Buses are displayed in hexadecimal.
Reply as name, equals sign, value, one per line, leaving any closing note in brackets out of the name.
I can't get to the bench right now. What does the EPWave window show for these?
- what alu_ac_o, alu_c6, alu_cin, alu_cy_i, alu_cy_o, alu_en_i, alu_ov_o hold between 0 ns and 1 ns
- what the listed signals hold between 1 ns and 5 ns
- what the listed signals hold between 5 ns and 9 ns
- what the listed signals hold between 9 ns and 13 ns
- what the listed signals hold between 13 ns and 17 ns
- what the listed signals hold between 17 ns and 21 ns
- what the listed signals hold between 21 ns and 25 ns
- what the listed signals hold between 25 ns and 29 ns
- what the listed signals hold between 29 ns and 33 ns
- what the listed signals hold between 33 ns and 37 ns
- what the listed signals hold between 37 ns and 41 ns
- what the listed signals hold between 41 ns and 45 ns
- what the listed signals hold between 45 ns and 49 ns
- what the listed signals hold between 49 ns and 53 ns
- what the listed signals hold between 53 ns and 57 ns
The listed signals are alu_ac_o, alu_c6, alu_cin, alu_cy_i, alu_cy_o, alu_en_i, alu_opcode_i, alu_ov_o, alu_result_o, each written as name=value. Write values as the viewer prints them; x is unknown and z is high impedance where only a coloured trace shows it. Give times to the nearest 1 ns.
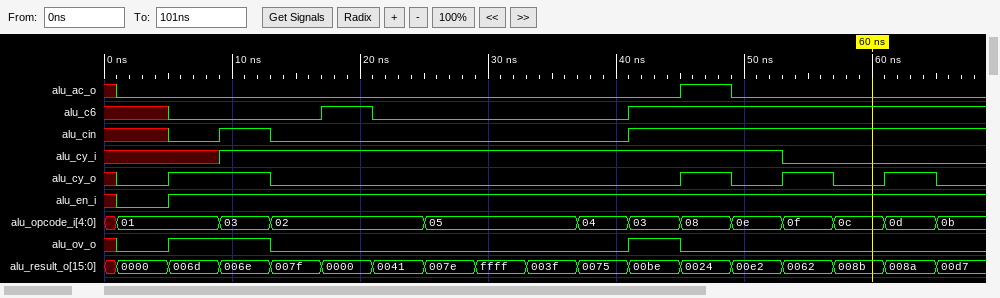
what alu_ac_o, alu_c6, alu_cin, alu_cy_i, alu_cy_o, alu_en_i, alu_ov_o hold between 0 ns and 1 ns = alu_ac_o=x, alu_c6=x, alu_cin=x, alu_cy_i=x, alu_cy_o=x, alu_en_i=x, alu_ov_o=x
what the listed signals hold between 1 ns and 5 ns = alu_ac_o=0, alu_c6=x, alu_cin=x, alu_cy_i=x, alu_cy_o=0, alu_en_i=0, alu_opcode_i=01, alu_ov_o=0, alu_result_o=0000
what the listed signals hold between 5 ns and 9 ns = alu_ac_o=0, alu_c6=0, alu_cin=0, alu_cy_i=x, alu_cy_o=1, alu_en_i=1, alu_opcode_i=01, alu_ov_o=1, alu_result_o=006d
what the listed signals hold between 9 ns and 13 ns = alu_ac_o=0, alu_c6=0, alu_cin=1, alu_cy_i=1, alu_cy_o=1, alu_en_i=1, alu_opcode_i=03, alu_ov_o=1, alu_result_o=006e
what the listed signals hold between 13 ns and 17 ns = alu_ac_o=0, alu_c6=0, alu_cin=0, alu_cy_i=1, alu_cy_o=0, alu_en_i=1, alu_opcode_i=02, alu_ov_o=0, alu_result_o=007f
what the listed signals hold between 17 ns and 21 ns = alu_ac_o=0, alu_c6=1, alu_cin=0, alu_cy_i=1, alu_cy_o=0, alu_en_i=1, alu_opcode_i=02, alu_ov_o=0, alu_result_o=0000
what the listed signals hold between 21 ns and 25 ns = alu_ac_o=0, alu_c6=0, alu_cin=0, alu_cy_i=1, alu_cy_o=0, alu_en_i=1, alu_opcode_i=02, alu_ov_o=0, alu_result_o=0041
what the listed signals hold between 25 ns and 29 ns = alu_ac_o=0, alu_c6=0, alu_cin=0, alu_cy_i=1, alu_cy_o=0, alu_en_i=1, alu_opcode_i=05, alu_ov_o=0, alu_result_o=007e
what the listed signals hold between 29 ns and 33 ns = alu_ac_o=0, alu_c6=0, alu_cin=0, alu_cy_i=1, alu_cy_o=0, alu_en_i=1, alu_opcode_i=05, alu_ov_o=0, alu_result_o=ffff
what the listed signals hold between 33 ns and 37 ns = alu_ac_o=0, alu_c6=0, alu_cin=0, alu_cy_i=1, alu_cy_o=0, alu_en_i=1, alu_opcode_i=05, alu_ov_o=0, alu_result_o=003f
what the listed signals hold between 37 ns and 41 ns = alu_ac_o=0, alu_c6=0, alu_cin=0, alu_cy_i=1, alu_cy_o=0, alu_en_i=1, alu_opcode_i=04, alu_ov_o=0, alu_result_o=0075
what the listed signals hold between 41 ns and 45 ns = alu_ac_o=0, alu_c6=1, alu_cin=1, alu_cy_i=1, alu_cy_o=0, alu_en_i=1, alu_opcode_i=03, alu_ov_o=1, alu_result_o=00be
what the listed signals hold between 45 ns and 49 ns = alu_ac_o=1, alu_c6=1, alu_cin=1, alu_cy_i=1, alu_cy_o=1, alu_en_i=1, alu_opcode_i=08, alu_ov_o=0, alu_result_o=0024
what the listed signals hold between 49 ns and 53 ns = alu_ac_o=0, alu_c6=1, alu_cin=1, alu_cy_i=1, alu_cy_o=0, alu_en_i=1, alu_opcode_i=0e, alu_ov_o=0, alu_result_o=00e2
what the listed signals hold between 53 ns and 57 ns = alu_ac_o=0, alu_c6=1, alu_cin=1, alu_cy_i=0, alu_cy_o=1, alu_en_i=1, alu_opcode_i=0f, alu_ov_o=0, alu_result_o=0062
